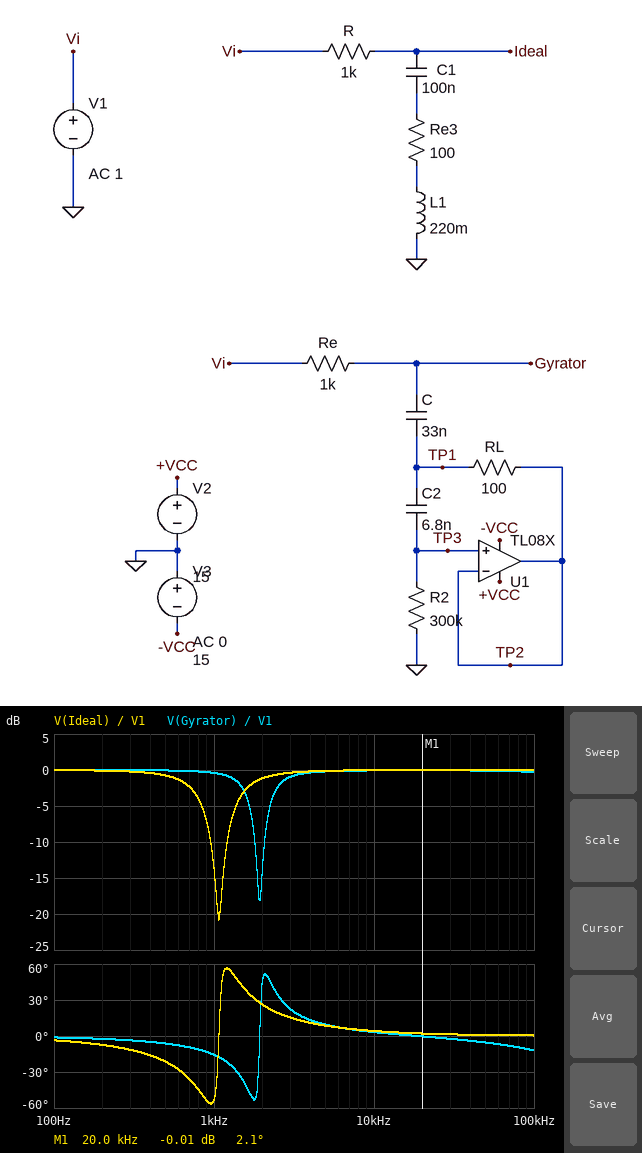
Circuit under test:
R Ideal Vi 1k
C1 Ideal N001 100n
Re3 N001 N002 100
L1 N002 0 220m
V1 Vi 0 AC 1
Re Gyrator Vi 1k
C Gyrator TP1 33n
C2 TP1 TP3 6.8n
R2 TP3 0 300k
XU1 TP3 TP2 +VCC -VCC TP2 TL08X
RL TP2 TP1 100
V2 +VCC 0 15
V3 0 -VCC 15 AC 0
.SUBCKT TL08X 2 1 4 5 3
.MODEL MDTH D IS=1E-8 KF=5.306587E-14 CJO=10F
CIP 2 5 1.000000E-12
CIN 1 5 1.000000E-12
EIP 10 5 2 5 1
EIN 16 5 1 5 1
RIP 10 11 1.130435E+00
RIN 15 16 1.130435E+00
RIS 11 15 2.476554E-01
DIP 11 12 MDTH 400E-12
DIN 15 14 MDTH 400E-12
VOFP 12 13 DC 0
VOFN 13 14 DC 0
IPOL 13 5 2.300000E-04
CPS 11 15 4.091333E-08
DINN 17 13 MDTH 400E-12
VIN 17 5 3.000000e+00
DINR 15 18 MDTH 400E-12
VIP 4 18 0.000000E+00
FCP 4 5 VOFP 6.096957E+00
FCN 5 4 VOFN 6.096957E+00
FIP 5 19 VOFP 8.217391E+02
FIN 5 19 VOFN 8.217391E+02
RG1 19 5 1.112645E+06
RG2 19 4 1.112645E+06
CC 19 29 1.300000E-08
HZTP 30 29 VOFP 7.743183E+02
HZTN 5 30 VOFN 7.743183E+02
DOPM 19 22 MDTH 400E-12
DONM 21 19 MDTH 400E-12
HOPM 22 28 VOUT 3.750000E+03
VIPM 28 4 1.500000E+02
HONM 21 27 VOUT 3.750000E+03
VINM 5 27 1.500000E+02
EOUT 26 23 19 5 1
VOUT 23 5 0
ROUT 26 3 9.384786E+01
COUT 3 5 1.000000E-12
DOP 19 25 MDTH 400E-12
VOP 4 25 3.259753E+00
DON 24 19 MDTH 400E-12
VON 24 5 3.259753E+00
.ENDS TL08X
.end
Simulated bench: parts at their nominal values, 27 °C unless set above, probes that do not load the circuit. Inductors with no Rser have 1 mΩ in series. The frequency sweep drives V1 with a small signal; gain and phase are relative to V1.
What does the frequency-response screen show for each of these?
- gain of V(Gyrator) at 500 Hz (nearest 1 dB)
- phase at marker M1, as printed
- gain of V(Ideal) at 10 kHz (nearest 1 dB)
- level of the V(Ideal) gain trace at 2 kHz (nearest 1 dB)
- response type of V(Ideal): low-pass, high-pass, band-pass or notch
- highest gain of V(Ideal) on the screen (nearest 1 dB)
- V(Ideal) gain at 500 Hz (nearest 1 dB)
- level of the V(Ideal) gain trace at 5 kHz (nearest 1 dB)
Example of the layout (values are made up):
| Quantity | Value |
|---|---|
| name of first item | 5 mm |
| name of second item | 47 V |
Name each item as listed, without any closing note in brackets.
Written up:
| Quantity | Value |
|---|---|
| gain of V(Gyrator) at 500 Hz | 0 dB |
| phase at marker M1, as printed | 2.1 deg |
| gain of V(Ideal) at 10 kHz | 0 dB |
| level of the V(Ideal) gain trace at 2 kHz | -1 dB |
| response type of V(Ideal): low-pass, high-pass, band-pass or notch | notch |
| highest gain of V(Ideal) on the screen | 0 dB |
| V(Ideal) gain at 500 Hz | -1 dB |
| level of the V(Ideal) gain trace at 5 kHz | 0 dB |
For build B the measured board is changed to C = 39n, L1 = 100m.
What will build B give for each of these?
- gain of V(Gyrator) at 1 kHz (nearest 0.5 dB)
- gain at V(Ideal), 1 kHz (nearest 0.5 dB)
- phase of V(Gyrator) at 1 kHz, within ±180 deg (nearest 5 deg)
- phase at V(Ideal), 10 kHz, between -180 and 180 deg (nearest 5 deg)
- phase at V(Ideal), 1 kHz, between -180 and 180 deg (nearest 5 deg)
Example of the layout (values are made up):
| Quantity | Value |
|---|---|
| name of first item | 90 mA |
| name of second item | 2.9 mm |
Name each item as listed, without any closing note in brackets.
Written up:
| Quantity | Value |
|---|---|
| gain of V(Gyrator) at 1 kHz | -0.5 dB |
| gain at V(Ideal), 1 kHz | -3.5 dB |
| phase of V(Gyrator) at 1 kHz, within ±180 deg | -20 deg |
| phase at V(Ideal), 10 kHz, between -180 and 180 deg | 10 deg |
| phase at V(Ideal), 1 kHz, between -180 and 180 deg | -45 deg |
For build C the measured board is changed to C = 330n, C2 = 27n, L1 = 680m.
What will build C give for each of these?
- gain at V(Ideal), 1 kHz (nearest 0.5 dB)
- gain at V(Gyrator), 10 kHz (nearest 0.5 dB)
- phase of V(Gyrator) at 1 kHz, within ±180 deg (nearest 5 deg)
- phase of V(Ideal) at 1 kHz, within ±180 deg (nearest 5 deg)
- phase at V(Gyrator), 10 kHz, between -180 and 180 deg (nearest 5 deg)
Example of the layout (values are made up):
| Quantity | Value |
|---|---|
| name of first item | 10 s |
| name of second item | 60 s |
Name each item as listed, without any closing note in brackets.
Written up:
| Quantity | Value |
|---|---|
| gain at V(Ideal), 1 kHz | -0.5 dB |
| gain at V(Gyrator), 10 kHz | 0 dB |
| phase of V(Gyrator) at 1 kHz, within ±180 deg | 10 deg |
| phase of V(Ideal) at 1 kHz, within ±180 deg | 20 deg |
| phase at V(Gyrator), 10 kHz, between -180 and 180 deg | 0 deg |
